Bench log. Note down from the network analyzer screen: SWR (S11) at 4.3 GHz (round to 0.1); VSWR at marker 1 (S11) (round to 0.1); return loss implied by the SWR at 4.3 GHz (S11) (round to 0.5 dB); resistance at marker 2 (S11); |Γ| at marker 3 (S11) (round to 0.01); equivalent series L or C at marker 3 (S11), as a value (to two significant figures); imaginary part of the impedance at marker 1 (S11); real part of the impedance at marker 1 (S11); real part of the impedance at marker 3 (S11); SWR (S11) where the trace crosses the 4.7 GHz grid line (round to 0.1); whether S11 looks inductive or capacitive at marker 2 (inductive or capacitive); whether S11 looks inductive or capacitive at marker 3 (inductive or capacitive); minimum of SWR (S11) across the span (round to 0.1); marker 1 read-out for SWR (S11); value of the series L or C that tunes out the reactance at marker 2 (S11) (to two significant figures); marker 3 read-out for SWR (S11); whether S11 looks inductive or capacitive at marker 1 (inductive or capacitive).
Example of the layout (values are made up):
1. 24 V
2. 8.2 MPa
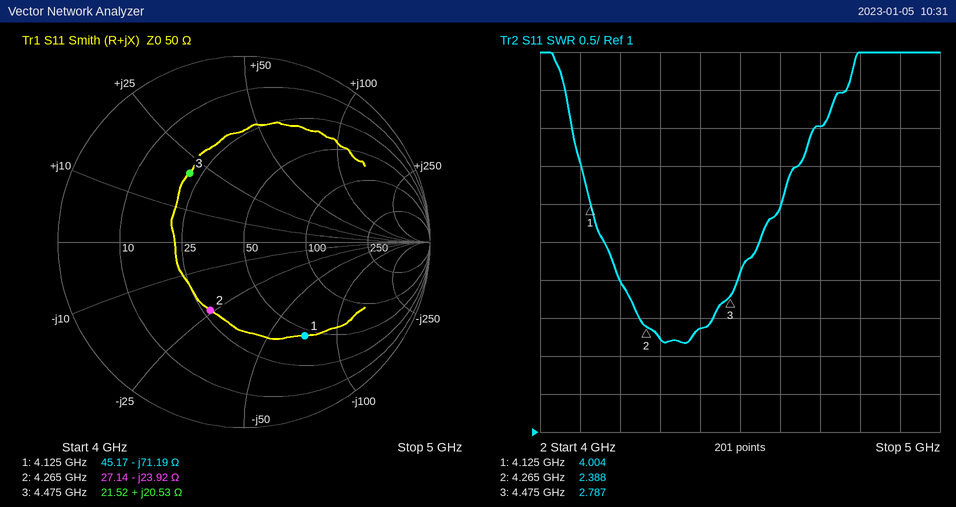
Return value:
1. 2.2
2. 4.0
3. 8.5 dB
4. 27.14 Ω
5. 0.47
6. 730 pH
7. -71.19 Ω
8. 45.17 Ω
9. 21.52 Ω
10. 5.0
11. capacitive
12. inductive
13. 2.2
14. 4.004
15. 890 pH
16. 2.787
17. capacitive
